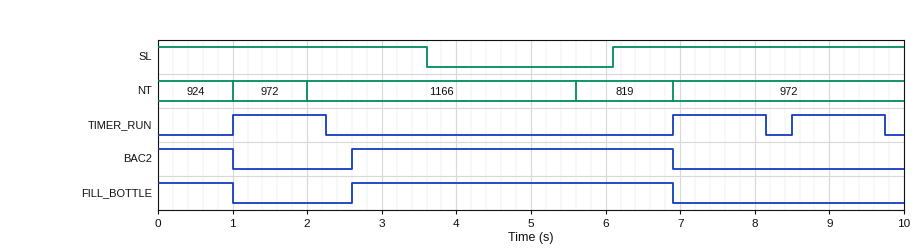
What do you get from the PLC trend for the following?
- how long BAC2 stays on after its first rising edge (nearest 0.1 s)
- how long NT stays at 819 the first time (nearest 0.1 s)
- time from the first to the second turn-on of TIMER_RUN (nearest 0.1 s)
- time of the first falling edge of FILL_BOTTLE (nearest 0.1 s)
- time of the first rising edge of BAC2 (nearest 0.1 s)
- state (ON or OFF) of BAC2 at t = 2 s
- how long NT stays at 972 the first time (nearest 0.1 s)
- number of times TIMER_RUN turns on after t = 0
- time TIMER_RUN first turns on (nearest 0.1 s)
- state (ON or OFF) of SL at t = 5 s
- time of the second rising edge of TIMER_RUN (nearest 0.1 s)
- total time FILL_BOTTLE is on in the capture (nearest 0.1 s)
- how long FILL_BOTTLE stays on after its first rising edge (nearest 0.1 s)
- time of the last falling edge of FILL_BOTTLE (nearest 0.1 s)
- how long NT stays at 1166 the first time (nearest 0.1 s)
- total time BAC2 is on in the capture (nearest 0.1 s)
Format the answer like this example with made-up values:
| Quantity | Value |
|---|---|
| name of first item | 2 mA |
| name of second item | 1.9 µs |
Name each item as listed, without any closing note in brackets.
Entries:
| Quantity | Value |
|---|---|
| how long BAC2 stays on after its first rising edge | 4.3 s |
| how long NT stays at 819 the first time | 1.3 s |
| time from the first to the second turn-on of TIMER_RUN | 5.9 s |
| time of the first falling edge of FILL_BOTTLE | 1.0 s |
| time of the first rising edge of BAC2 | 2.6 s |
| state (ON or OFF) of BAC2 at t = 2 s | OFF |
| how long NT stays at 972 the first time | 1.0 s |
| number of times TIMER_RUN turns on after t = 0 | 3 |
| time TIMER_RUN first turns on | 1.0 s |
| state (ON or OFF) of SL at t = 5 s | OFF |
| time of the second rising edge of TIMER_RUN | 6.9 s |
| total time FILL_BOTTLE is on in the capture | 5.3 s |
| how long FILL_BOTTLE stays on after its first rising edge | 4.3 s |
| time of the last falling edge of FILL_BOTTLE | 6.9 s |
| how long NT stays at 1166 the first time | 3.6 s |
| total time BAC2 is on in the capture | 5.3 s |
